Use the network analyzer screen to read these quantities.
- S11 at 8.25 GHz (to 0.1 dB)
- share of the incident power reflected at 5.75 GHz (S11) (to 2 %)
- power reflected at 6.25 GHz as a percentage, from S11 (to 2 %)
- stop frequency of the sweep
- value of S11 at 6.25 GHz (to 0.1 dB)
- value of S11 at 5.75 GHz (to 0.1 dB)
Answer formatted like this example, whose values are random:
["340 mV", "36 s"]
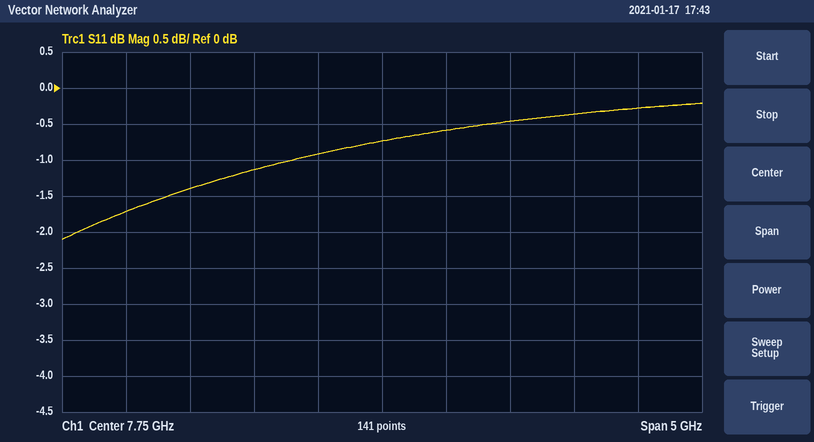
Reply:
["-0.6 dB", "68 %", "72 %", "10.25 GHz", "-1.4 dB", "-1.7 dB"]
